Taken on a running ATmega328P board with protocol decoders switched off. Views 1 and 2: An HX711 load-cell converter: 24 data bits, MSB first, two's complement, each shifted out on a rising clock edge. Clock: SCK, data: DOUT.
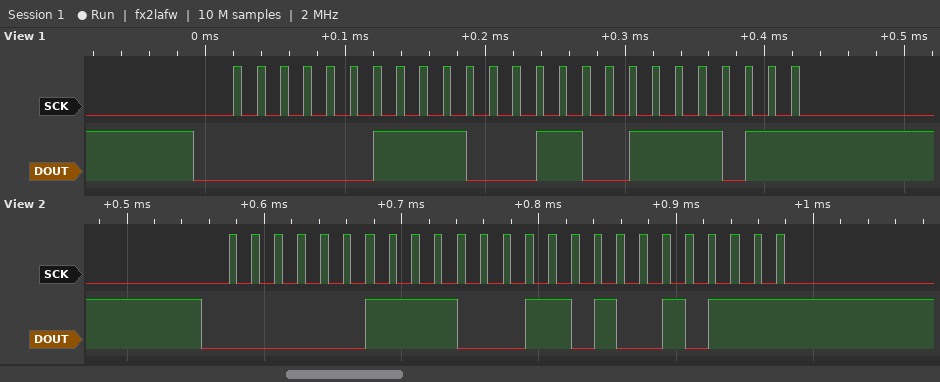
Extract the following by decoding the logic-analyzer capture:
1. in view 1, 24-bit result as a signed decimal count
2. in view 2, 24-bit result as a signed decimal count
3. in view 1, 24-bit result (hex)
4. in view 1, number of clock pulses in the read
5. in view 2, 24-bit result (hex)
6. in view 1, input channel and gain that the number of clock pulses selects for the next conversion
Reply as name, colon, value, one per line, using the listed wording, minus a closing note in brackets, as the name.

in view 1, 24-bit result as a signed decimal count: 247419
in view 2, 24-bit result as a signed decimal count: 247447
in view 1, 24-bit result: 0x03C67B
in view 1, number of clock pulses in the read: 25
in view 2, 24-bit result: 0x03C697
in view 1, input channel and gain that the number of clock pulses selects for the next conversion: channel A, gain 128
